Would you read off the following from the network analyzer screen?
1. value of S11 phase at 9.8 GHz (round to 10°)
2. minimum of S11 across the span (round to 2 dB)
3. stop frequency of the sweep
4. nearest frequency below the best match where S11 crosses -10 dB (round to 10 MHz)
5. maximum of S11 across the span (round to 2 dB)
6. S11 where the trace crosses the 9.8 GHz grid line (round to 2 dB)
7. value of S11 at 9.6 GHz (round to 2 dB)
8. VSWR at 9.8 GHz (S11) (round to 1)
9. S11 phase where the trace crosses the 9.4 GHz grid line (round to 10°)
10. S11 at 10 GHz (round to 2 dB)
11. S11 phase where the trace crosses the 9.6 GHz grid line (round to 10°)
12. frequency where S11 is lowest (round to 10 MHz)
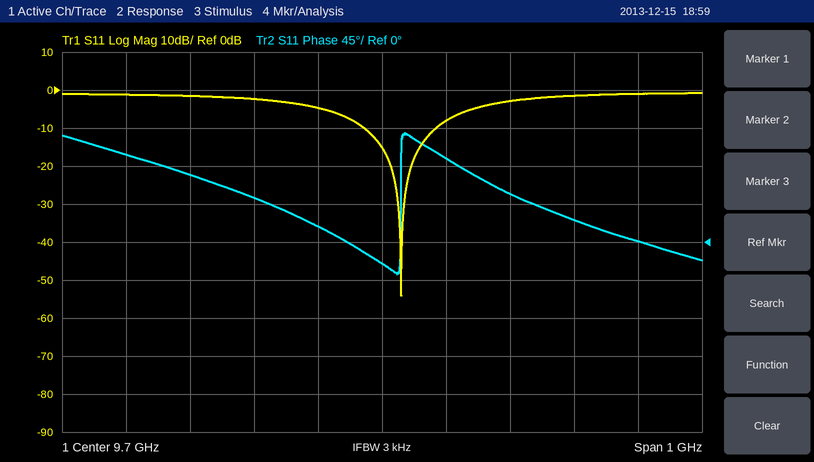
100°
-54 dB
10.2 GHz
9.67 GHz
0 dB
-8 dB
-4 dB
2
80°
-2 dB
20°
9.73 GHz
